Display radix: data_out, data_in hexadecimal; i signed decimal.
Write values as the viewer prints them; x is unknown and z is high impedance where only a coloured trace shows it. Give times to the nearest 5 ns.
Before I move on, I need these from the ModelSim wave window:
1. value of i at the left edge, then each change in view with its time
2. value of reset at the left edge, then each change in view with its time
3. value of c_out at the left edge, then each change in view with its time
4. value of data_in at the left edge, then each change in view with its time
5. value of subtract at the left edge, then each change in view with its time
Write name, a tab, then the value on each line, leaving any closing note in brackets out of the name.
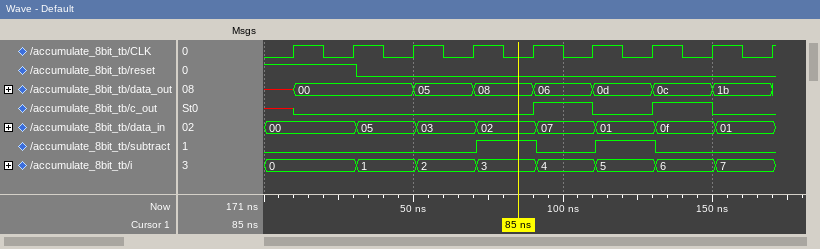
value of i at the left edge, then each change in view with its time	0, 1 at 30 ns, 2 at 50 ns, 3 at 70 ns, 4 at 90 ns, 5 at 110 ns, 6 at 130 ns, 7 at 150 ns
value of reset at the left edge, then each change in view with its time	1, 0 at 30 ns
value of c_out at the left edge, then each change in view with its time	x, 0 at 10 ns, 1 at 90 ns, 0 at 110 ns, 1 at 130 ns, 0 at 150 ns
value of data_in at the left edge, then each change in view with its time	00, 05 at 30 ns, 03 at 50 ns, 02 at 70 ns, 07 at 90 ns, 01 at 110 ns, 0f at 130 ns, 01 at 150 ns
value of subtract at the left edge, then each change in view with its time	0, 1 at 70 ns, 0 at 90 ns, 1 at 110 ns, 0 at 130 ns
